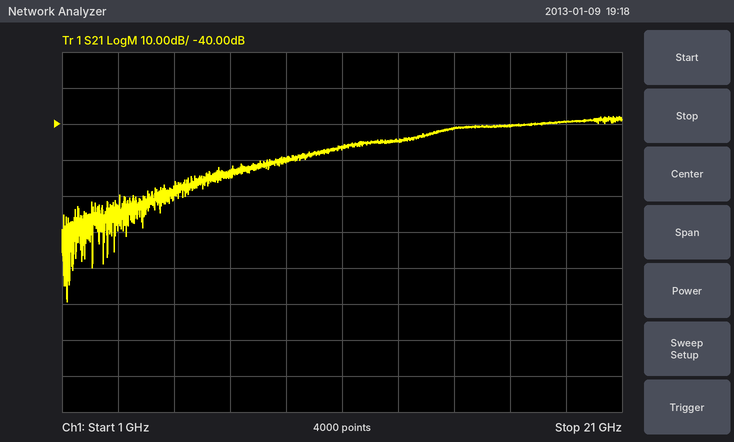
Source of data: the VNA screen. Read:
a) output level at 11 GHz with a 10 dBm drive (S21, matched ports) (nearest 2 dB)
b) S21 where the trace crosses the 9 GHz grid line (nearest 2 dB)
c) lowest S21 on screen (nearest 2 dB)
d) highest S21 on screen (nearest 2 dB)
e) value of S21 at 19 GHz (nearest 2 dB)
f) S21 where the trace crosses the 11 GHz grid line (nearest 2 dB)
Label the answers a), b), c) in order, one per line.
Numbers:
a) -36 dBm
b) -50 dB
c) -90 dB
d) -38 dB
e) -40 dB
f) -46 dB
